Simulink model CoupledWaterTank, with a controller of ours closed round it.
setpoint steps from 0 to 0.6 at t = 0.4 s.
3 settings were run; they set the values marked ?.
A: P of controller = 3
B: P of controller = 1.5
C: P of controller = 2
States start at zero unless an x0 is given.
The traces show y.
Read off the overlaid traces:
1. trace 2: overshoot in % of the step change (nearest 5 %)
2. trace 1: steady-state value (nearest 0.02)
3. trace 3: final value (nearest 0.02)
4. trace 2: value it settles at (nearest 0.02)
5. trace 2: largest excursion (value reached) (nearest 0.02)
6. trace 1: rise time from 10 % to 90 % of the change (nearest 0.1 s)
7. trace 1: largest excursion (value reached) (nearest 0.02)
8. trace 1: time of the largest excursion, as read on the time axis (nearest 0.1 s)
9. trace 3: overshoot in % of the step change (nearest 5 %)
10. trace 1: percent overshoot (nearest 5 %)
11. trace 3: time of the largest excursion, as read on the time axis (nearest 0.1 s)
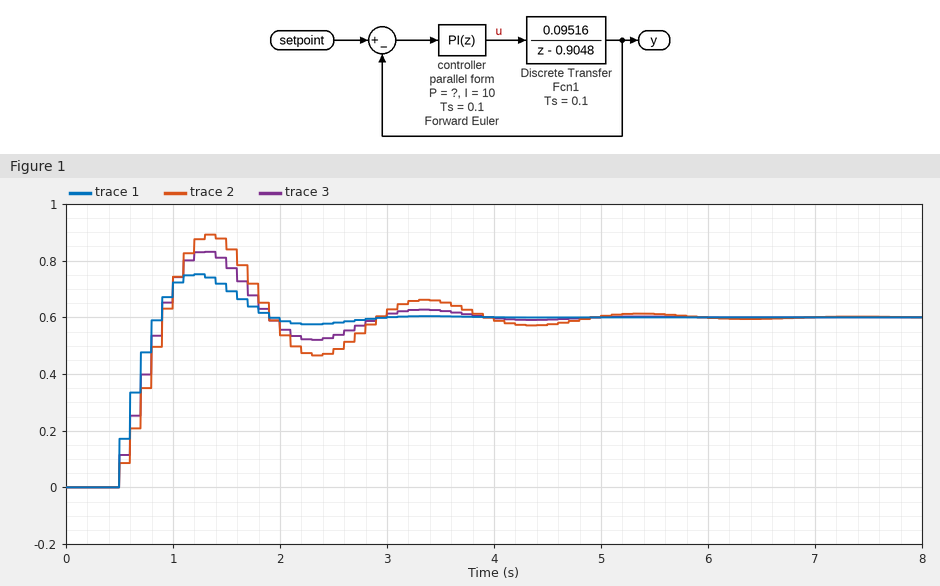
50 %
0.60
0.60
0.60
0.90
0.3 s
0.76
1.2 s
40 %
25 %
1.3 s
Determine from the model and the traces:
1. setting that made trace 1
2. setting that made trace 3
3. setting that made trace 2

A
C
B
